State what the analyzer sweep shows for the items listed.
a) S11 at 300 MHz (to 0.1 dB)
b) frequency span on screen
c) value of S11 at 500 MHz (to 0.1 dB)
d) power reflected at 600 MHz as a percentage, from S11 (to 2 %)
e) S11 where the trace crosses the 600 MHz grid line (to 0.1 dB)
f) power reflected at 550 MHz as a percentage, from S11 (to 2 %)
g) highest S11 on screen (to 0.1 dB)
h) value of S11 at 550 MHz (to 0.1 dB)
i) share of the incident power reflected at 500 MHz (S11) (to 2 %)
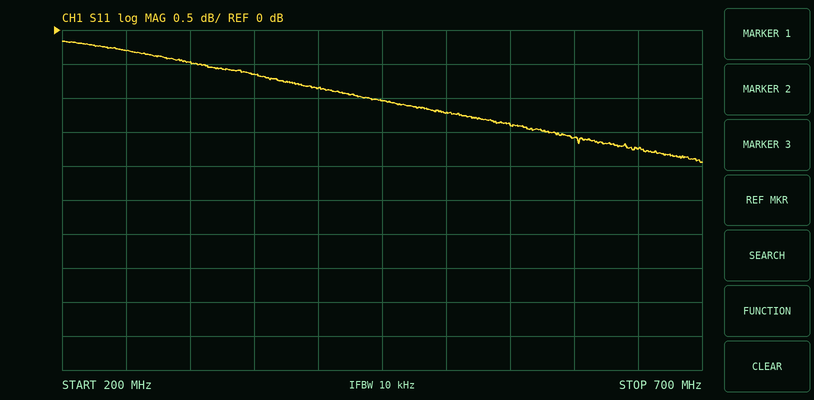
-0.5 dB
500 MHz
-1.2 dB
70 %
-1.6 dB
72 %
-0.2 dB
-1.4 dB
76 %
